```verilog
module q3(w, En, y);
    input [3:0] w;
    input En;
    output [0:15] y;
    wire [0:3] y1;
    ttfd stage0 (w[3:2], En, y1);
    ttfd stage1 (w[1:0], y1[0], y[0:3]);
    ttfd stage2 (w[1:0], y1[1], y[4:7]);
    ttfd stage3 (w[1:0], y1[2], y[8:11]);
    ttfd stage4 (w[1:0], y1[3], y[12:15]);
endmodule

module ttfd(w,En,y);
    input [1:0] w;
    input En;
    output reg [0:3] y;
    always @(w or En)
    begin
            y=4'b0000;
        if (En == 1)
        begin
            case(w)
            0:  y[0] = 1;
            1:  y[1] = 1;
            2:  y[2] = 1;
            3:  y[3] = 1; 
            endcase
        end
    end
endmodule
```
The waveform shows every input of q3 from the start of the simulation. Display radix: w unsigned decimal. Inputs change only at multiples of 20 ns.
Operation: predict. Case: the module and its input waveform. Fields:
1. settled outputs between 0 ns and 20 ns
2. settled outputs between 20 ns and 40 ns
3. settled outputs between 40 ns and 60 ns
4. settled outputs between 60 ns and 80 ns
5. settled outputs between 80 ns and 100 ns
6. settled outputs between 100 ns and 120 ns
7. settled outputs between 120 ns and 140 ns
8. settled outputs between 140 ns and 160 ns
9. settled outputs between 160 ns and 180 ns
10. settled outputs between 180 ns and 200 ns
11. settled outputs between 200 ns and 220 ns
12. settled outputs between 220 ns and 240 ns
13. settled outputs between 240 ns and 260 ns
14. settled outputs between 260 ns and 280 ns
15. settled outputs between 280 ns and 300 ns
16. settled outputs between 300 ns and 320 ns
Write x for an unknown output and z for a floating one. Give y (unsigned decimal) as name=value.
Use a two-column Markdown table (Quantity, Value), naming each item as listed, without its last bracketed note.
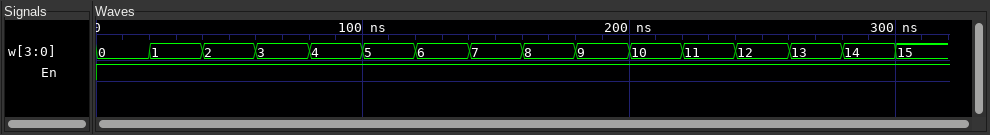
| Quantity | Value |
|---|---|
| settled outputs between 0 ns and 20 ns | y=32768 |
| settled outputs between 20 ns and 40 ns | y=16384 |
| settled outputs between 40 ns and 60 ns | y=8192 |
| settled outputs between 60 ns and 80 ns | y=4096 |
| settled outputs between 80 ns and 100 ns | y=2048 |
| settled outputs between 100 ns and 120 ns | y=1024 |
| settled outputs between 120 ns and 140 ns | y=512 |
| settled outputs between 140 ns and 160 ns | y=256 |
| settled outputs between 160 ns and 180 ns | y=128 |
| settled outputs between 180 ns and 200 ns | y=64 |
| settled outputs between 200 ns and 220 ns | y=32 |
| settled outputs between 220 ns and 240 ns | y=16 |
| settled outputs between 240 ns and 260 ns | y=8 |
| settled outputs between 260 ns and 280 ns | y=4 |
| settled outputs between 280 ns and 300 ns | y=2 |
| settled outputs between 300 ns and 320 ns | y=1 |
